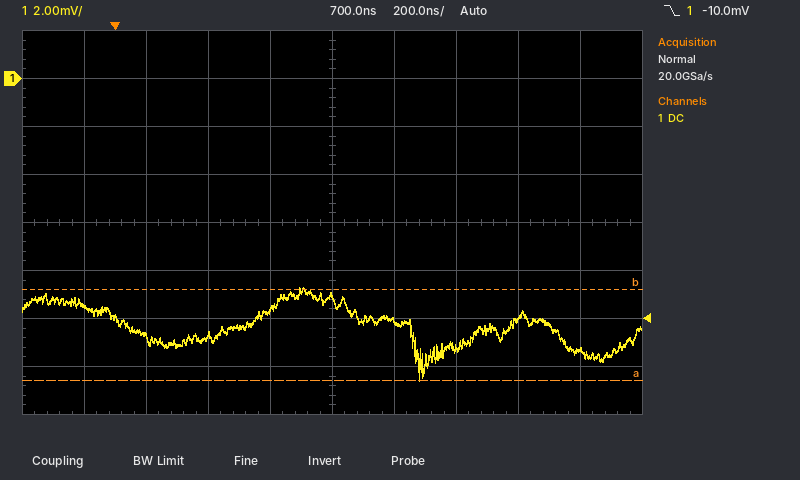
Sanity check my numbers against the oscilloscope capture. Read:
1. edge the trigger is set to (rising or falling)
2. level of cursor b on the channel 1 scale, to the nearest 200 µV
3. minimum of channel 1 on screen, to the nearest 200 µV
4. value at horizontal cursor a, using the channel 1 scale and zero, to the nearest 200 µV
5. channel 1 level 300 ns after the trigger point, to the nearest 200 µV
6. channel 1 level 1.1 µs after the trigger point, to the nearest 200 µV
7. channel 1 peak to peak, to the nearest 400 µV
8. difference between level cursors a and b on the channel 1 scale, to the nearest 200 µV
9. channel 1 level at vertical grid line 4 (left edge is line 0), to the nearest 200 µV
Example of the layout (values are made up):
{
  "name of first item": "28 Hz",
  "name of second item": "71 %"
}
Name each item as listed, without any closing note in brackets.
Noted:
{
  "edge the trigger is set to": "falling",
  "level of cursor b on the channel 1 scale, to the nearest 200 µV": "-8.8 mV",
  "minimum of channel 1 on screen, to the nearest 200 µV": "-12.6 mV",
  "value at horizontal cursor a, using the channel 1 scale and zero, to the nearest 200 µV": "-12.6 mV",
  "channel 1 level 300 ns after the trigger point, to the nearest 200 µV": "-10.8 mV",
  "channel 1 level 1.1 µs after the trigger point, to the nearest 200 µV": "-11.2 mV",
  "channel 1 peak to peak, to the nearest 400 µV": "4.0 mV",
  "difference between level cursors a and b on the channel 1 scale, to the nearest 200 µV": "3.8 mV",
  "channel 1 level at vertical grid line 4 (left edge is line 0), to the nearest 200 µV": "-9.6 mV"
}
